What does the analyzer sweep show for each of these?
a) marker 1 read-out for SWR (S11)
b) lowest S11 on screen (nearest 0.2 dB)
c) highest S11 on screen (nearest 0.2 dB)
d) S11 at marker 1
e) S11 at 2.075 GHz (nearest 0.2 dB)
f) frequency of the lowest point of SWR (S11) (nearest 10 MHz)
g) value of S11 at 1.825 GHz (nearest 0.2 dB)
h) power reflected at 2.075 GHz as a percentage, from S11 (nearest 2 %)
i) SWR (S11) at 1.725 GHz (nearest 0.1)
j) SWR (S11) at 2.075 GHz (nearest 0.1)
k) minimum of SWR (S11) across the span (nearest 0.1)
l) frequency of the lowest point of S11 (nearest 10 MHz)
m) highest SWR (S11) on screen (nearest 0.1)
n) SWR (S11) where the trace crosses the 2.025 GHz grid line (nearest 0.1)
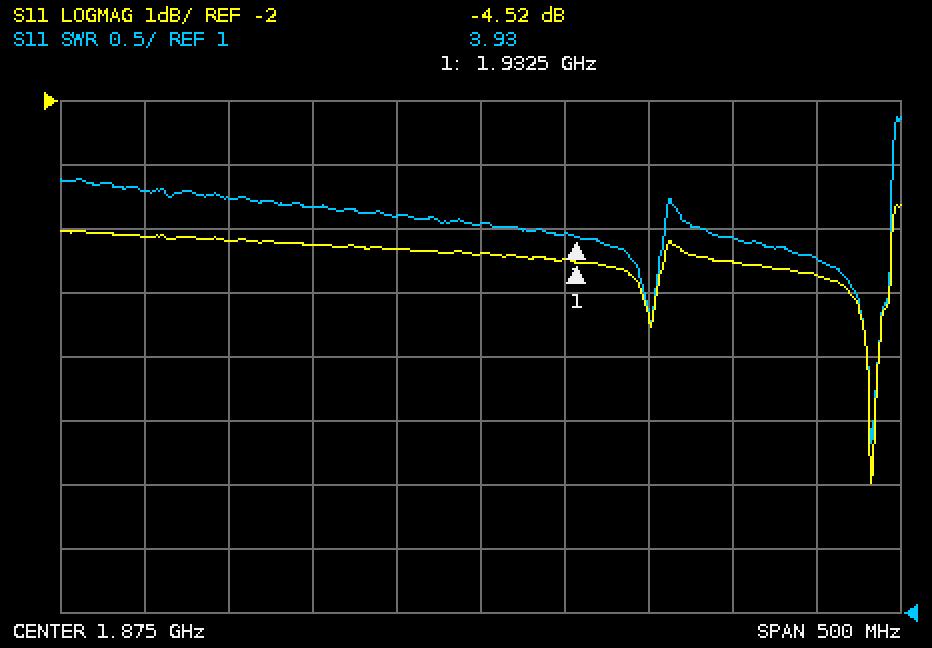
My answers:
3.93
-8.0 dB
-3.6 dB
-4.52 dB
-4.8 dB
2.11 GHz
-4.4 dB
34 %
4.2
3.8
2.3
2.11 GHz
4.9
3.9
